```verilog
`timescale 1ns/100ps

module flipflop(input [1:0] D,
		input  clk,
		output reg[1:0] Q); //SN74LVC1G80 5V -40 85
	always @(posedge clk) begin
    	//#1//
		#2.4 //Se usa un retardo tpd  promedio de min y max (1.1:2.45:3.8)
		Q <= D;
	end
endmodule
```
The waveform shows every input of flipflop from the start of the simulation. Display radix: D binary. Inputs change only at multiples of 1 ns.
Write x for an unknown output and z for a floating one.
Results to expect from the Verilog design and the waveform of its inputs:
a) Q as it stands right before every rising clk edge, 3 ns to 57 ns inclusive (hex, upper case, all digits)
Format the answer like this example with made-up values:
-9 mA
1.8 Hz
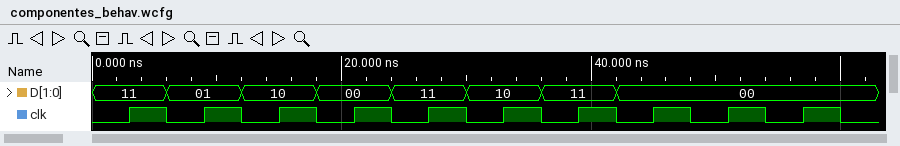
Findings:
x, 3, 1, 2, 0, 3, 2, 3, 0, 0
